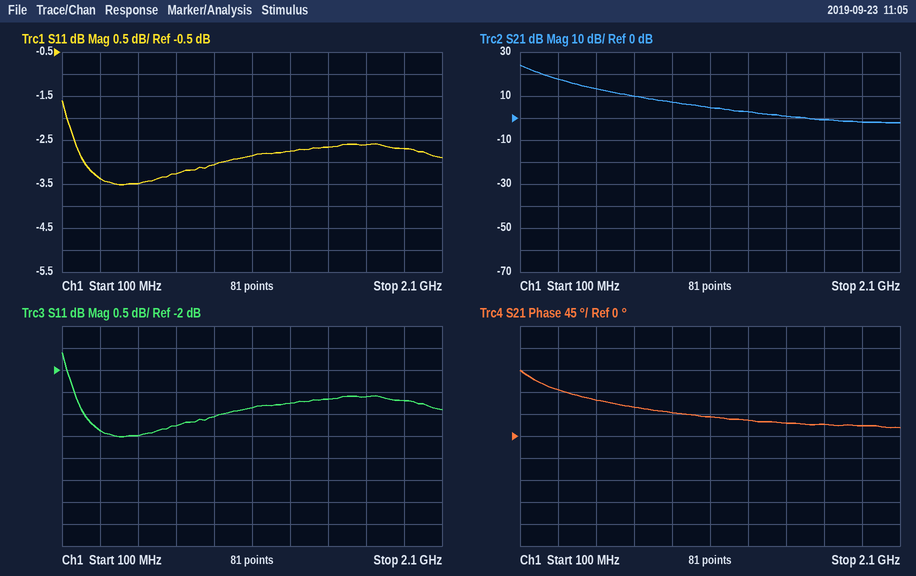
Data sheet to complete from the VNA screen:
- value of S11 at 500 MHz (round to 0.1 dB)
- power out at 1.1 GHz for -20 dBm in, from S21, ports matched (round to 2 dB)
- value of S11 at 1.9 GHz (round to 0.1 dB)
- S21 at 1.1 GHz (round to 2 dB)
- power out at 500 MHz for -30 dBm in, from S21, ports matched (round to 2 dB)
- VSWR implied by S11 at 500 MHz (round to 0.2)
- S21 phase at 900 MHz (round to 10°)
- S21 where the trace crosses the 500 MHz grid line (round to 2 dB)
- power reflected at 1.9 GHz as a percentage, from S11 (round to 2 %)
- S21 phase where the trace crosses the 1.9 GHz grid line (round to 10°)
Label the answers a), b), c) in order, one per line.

a) -3.5 dB
b) -16 dBm
c) -2.7 dB
d) 4 dB
e) -16 dBm
f) 5.0
g) 50°
h) 14 dB
i) 54 %
j) 20°
